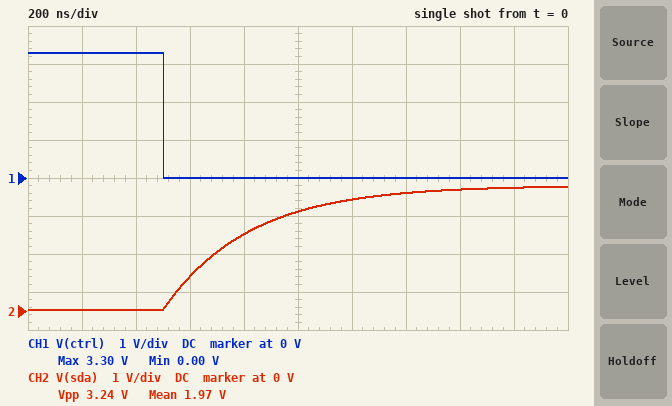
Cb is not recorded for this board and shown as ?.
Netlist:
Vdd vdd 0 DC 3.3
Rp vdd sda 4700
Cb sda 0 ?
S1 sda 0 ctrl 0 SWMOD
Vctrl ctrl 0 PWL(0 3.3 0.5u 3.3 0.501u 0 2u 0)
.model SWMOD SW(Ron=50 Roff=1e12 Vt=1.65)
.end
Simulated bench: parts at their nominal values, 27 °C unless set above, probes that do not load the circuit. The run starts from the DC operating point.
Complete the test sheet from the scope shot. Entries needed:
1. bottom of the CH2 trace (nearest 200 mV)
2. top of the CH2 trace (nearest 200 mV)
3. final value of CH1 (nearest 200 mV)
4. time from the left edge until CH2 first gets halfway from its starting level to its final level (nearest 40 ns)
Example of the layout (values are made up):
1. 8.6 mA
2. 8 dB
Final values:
1. 0 V
2. 3.2 V
3. 0 V
4. 720 ns
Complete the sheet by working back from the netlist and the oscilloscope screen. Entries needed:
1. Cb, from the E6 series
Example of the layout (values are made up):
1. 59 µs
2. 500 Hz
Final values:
1. 68 pF
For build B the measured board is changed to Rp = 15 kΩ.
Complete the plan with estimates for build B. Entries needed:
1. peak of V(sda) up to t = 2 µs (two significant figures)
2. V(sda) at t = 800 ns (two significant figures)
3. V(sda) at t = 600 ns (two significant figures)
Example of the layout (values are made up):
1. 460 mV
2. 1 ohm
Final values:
1. 2.5 V
2. 850 mV
3. 320 mV
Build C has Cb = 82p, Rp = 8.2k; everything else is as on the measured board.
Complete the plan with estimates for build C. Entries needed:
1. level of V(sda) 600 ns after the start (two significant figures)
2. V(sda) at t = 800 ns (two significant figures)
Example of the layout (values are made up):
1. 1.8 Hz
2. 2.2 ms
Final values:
1. 470 mV
2. 1.2 V
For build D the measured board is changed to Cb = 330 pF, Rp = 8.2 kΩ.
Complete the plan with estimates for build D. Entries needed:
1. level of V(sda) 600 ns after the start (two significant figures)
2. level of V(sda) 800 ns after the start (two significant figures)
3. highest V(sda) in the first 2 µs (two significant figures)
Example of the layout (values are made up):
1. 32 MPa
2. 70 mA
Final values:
1. 140 mV
2. 360 mV
3. 1.4 V
